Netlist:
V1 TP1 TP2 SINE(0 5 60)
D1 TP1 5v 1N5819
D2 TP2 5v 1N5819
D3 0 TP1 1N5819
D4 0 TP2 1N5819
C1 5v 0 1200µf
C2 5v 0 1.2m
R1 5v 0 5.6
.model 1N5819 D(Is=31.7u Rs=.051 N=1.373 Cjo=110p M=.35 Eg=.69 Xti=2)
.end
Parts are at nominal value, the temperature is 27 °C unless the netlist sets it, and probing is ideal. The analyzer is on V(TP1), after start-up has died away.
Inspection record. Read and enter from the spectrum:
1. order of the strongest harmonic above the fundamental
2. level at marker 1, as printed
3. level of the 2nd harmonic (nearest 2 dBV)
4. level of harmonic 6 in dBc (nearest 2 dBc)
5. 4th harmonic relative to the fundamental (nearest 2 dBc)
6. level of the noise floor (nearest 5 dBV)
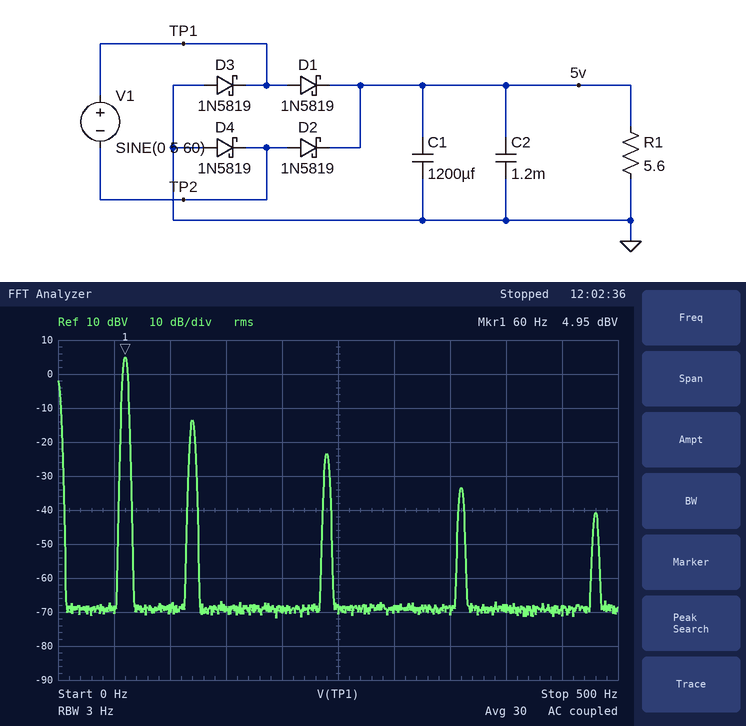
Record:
2
4.95 dBV
-14 dBV
-38 dBc
-28 dBc
-70 dBV
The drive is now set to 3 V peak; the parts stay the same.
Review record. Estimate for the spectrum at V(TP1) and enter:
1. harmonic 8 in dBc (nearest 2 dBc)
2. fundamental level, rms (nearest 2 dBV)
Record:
-48 dBc
0 dBV
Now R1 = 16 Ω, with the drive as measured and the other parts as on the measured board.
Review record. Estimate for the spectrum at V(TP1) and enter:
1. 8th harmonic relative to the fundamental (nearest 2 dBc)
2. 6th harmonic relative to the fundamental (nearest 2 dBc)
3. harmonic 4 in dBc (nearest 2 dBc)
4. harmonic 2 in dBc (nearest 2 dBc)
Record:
-48 dBc
-40 dBc
-34 dBc
-26 dBc
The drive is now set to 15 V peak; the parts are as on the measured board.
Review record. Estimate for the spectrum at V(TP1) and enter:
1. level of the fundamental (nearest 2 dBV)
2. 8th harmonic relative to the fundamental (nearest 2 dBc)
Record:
14 dBV
-44 dBc
